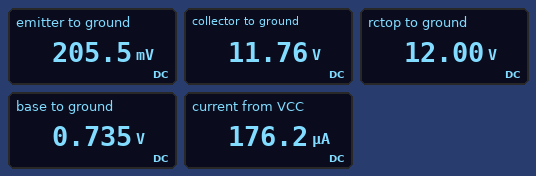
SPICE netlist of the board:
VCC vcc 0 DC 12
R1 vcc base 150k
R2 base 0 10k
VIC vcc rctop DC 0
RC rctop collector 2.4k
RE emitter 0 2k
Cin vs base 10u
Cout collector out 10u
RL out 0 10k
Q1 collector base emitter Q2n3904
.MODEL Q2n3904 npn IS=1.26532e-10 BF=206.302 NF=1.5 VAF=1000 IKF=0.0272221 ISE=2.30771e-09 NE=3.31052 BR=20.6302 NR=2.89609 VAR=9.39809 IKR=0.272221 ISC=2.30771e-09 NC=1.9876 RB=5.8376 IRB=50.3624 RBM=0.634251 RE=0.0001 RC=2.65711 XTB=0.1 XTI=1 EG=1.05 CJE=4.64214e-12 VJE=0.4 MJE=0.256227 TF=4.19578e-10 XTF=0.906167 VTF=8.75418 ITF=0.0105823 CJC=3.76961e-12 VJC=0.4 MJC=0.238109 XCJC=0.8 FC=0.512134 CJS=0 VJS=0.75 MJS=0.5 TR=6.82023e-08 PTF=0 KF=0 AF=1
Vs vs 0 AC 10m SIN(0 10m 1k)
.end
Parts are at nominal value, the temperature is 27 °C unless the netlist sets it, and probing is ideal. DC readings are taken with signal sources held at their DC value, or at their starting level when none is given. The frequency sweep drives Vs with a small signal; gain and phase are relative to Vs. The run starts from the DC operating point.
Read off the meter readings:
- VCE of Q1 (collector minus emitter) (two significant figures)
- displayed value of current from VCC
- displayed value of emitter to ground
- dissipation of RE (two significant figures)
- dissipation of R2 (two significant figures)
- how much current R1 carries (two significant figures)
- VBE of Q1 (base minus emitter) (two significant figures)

12 V
176.2 µA
205.5 mV
21 µW
54 µW
75 µA
530 mV
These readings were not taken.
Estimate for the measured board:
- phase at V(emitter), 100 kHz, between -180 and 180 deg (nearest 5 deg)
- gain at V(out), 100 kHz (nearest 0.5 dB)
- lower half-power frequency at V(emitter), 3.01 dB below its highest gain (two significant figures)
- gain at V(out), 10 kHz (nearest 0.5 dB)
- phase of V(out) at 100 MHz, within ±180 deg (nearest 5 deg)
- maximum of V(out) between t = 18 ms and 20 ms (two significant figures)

0 deg
-2.0 dB
2.7 Hz
-2.0 dB
30 deg
8.0 mV
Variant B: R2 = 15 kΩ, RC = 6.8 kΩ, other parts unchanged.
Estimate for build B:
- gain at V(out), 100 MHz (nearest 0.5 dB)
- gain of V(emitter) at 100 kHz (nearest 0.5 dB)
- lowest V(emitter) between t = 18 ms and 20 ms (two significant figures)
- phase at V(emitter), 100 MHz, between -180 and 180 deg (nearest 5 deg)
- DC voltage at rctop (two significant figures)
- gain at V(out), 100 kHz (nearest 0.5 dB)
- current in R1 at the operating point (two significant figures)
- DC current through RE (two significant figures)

1.5 dB
-0.5 dB
480 mV
0 deg
12 V
5.5 dB
73 µA
240 µA
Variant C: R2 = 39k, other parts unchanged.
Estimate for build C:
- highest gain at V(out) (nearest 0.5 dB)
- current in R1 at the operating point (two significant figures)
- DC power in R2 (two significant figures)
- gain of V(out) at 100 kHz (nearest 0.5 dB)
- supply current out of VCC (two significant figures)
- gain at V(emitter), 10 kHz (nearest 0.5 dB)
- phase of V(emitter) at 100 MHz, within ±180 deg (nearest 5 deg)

1.0 dB
65 µA
130 µW
-0.5 dB
880 µA
0 dB
0 deg
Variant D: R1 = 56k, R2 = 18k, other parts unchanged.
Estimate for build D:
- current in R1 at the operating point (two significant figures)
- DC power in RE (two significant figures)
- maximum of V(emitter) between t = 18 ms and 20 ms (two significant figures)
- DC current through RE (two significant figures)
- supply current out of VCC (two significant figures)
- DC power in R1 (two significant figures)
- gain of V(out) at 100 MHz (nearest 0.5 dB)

160 µA
2.4 mW
2.2 V
1.1 mA
1.2 mA
1.5 mW
1.0 dB
